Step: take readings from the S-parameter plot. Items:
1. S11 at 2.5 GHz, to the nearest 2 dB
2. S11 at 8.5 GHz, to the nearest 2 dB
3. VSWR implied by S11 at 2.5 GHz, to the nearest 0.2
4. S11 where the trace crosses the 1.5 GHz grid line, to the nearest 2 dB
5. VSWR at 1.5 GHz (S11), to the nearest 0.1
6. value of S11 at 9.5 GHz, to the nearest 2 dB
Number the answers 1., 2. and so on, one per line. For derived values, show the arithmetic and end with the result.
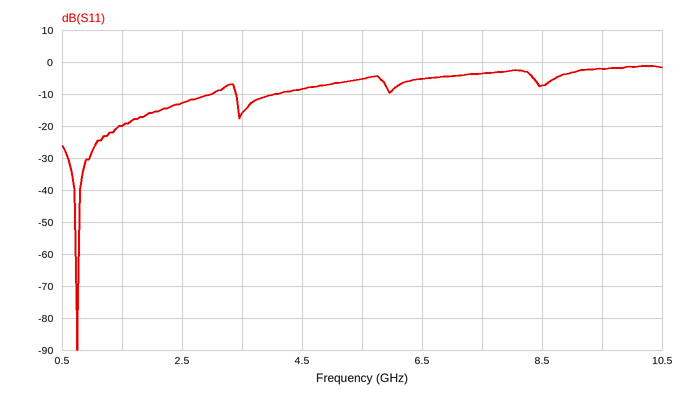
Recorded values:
1. -12 dB
2. -8 dB
3. |Γ| = 10^(-12/20) = 0.2512; VSWR = (1 + 0.2512)/(1 − 0.2512) ≈ 1.67, so 1.6 to the nearest 0.2
4. -20 dB
5. |Γ| = 10^(-20/20) = 0.1000; VSWR = (1 + 0.1000)/(1 − 0.1000) ≈ 1.2
6. -2 dB
